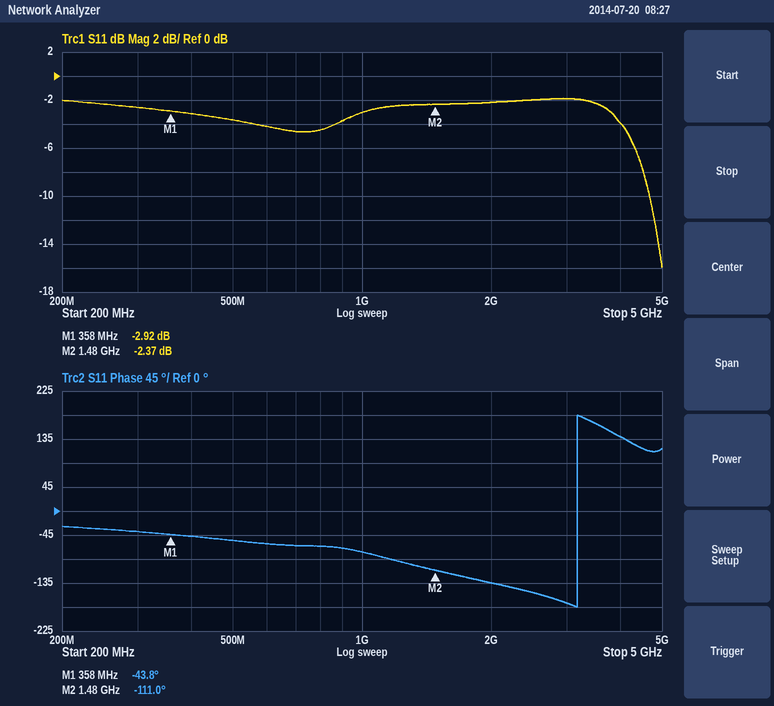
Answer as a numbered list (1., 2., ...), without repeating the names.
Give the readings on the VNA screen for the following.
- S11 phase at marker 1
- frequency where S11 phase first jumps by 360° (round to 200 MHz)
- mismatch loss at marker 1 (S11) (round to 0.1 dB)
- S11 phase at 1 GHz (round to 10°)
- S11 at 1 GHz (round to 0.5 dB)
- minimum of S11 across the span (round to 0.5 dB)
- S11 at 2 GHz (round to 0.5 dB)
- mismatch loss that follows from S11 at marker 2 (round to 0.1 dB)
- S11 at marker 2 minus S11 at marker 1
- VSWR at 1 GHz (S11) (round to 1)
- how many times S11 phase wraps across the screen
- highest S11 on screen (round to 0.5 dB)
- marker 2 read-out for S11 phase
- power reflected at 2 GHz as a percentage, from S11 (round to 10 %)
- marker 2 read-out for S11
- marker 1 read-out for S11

1. -43.8°
2. 3.2 GHz
3. 3.1 dB
4. -80°
5. -3.0 dB
6. -16.0 dB
7. -2.0 dB
8. 3.8 dB
9. 0.55 dB
10. 6
11. 1
12. -2.0 dB
13. -111.0°
14. 60 %
15. -2.37 dB
16. -2.92 dB
